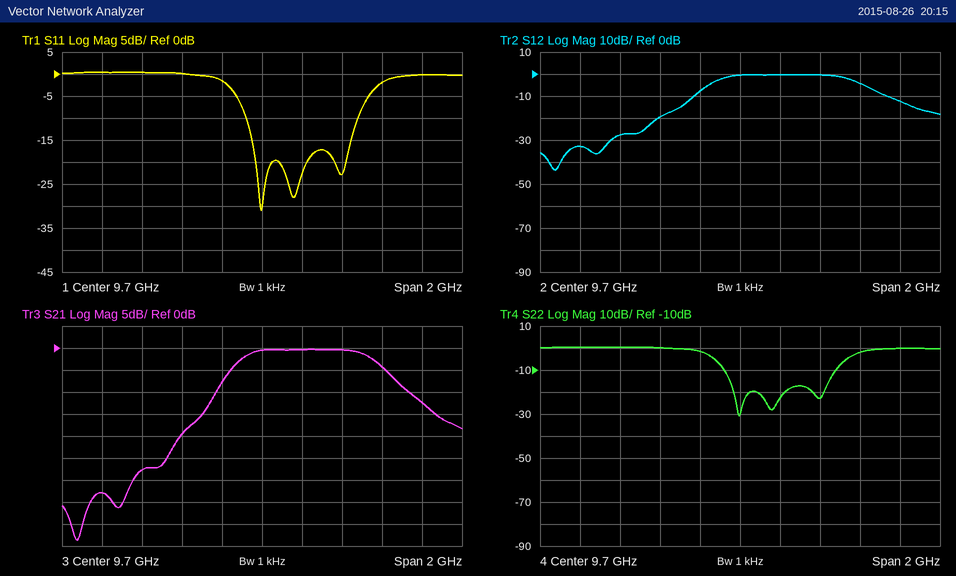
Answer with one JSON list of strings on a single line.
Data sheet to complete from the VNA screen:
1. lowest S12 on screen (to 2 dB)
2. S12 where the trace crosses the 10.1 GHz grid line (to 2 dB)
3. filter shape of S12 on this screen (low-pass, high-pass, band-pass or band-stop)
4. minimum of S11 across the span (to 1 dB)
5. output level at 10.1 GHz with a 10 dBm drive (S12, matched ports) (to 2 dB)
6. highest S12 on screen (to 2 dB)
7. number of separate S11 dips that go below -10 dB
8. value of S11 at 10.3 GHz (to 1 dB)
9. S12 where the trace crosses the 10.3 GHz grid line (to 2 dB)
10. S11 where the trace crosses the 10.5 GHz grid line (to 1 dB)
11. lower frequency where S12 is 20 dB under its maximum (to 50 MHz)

["-44 dB", "0 dB", "band-pass", "-31 dB", "10 dBm", "0 dB", "3", "-2 dB", "-4 dB", "0 dB", "9.30 GHz"]
